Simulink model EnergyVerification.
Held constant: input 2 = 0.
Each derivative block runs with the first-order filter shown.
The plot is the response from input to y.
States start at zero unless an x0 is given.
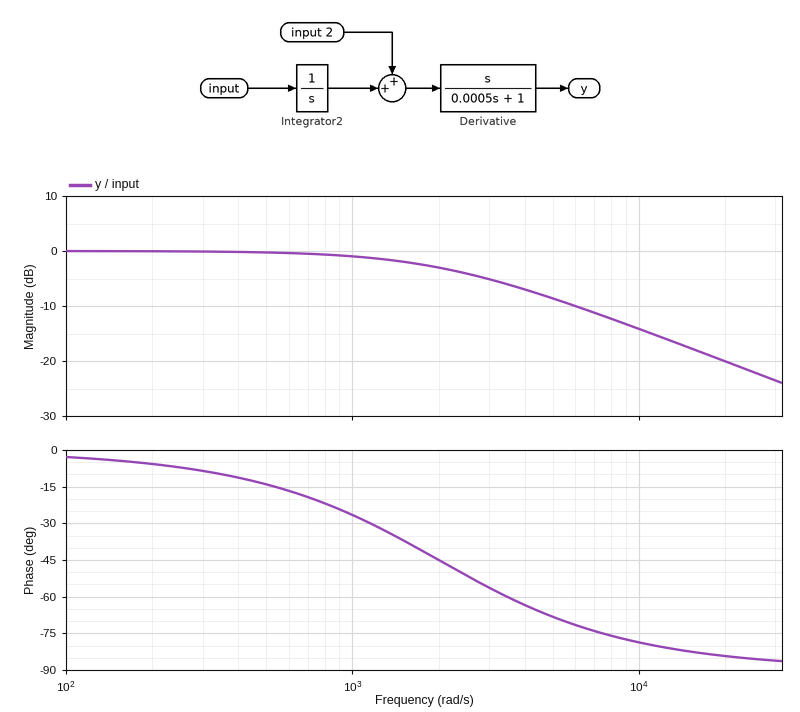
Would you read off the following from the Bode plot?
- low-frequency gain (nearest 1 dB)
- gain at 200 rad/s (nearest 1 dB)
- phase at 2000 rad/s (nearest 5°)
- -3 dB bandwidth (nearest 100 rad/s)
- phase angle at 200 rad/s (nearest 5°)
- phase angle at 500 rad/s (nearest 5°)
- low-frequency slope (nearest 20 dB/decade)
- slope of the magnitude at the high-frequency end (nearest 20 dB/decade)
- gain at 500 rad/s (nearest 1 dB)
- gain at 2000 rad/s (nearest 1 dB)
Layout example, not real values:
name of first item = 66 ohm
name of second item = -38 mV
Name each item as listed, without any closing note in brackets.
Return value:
low-frequency gain = 0 dB
gain at 200 rad/s = 0 dB
phase at 2000 rad/s = -45°
-3 dB bandwidth = 2000 rad/s
phase angle at 200 rad/s = -5°
phase angle at 500 rad/s = -15°
low-frequency slope = 0 dB/decade
slope of the magnitude at the high-frequency end = -20 dB/decade
gain at 500 rad/s = 0 dB
gain at 2000 rad/s = -3 dB
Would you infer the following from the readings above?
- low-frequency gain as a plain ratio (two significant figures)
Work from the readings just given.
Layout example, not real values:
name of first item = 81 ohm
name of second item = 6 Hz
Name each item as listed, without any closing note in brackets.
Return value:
low-frequency gain as a plain ratio = 1.0
